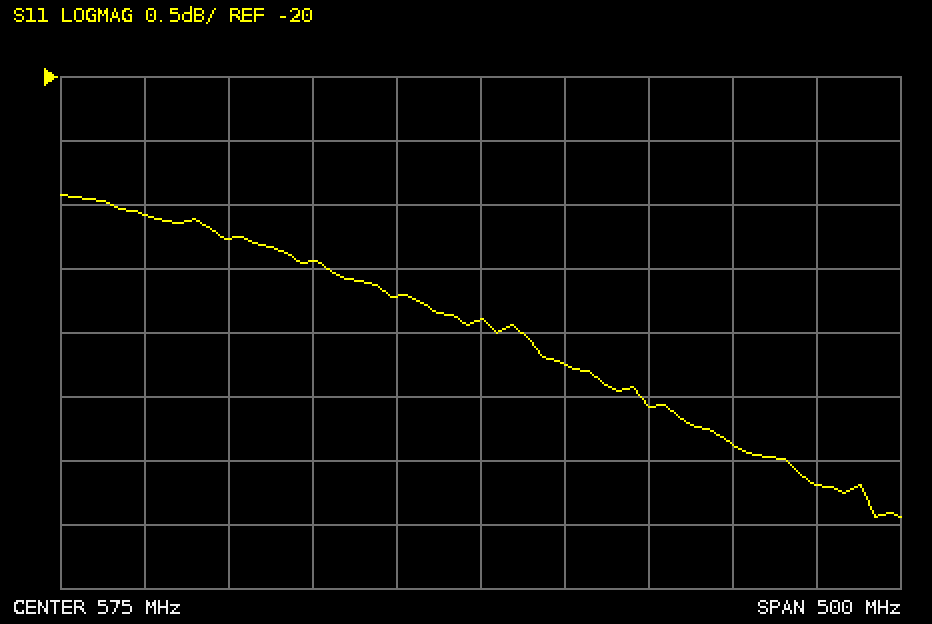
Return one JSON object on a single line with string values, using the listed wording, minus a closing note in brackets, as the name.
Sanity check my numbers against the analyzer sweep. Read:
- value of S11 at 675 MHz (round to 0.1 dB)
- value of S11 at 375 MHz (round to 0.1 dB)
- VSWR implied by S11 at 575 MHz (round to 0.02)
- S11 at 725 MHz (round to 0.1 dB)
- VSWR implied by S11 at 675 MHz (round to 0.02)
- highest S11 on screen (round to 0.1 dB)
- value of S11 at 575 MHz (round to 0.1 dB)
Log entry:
{"value of S11 at 675 MHz": "-22.6 dB", "value of S11 at 375 MHz": "-21.1 dB", "VSWR implied by S11 at 575 MHz": "1.18", "S11 at 725 MHz": "-22.9 dB", "VSWR implied by S11 at 675 MHz": "1.16", "highest S11 on screen": "-20.9 dB", "value of S11 at 575 MHz": "-21.9 dB"}
